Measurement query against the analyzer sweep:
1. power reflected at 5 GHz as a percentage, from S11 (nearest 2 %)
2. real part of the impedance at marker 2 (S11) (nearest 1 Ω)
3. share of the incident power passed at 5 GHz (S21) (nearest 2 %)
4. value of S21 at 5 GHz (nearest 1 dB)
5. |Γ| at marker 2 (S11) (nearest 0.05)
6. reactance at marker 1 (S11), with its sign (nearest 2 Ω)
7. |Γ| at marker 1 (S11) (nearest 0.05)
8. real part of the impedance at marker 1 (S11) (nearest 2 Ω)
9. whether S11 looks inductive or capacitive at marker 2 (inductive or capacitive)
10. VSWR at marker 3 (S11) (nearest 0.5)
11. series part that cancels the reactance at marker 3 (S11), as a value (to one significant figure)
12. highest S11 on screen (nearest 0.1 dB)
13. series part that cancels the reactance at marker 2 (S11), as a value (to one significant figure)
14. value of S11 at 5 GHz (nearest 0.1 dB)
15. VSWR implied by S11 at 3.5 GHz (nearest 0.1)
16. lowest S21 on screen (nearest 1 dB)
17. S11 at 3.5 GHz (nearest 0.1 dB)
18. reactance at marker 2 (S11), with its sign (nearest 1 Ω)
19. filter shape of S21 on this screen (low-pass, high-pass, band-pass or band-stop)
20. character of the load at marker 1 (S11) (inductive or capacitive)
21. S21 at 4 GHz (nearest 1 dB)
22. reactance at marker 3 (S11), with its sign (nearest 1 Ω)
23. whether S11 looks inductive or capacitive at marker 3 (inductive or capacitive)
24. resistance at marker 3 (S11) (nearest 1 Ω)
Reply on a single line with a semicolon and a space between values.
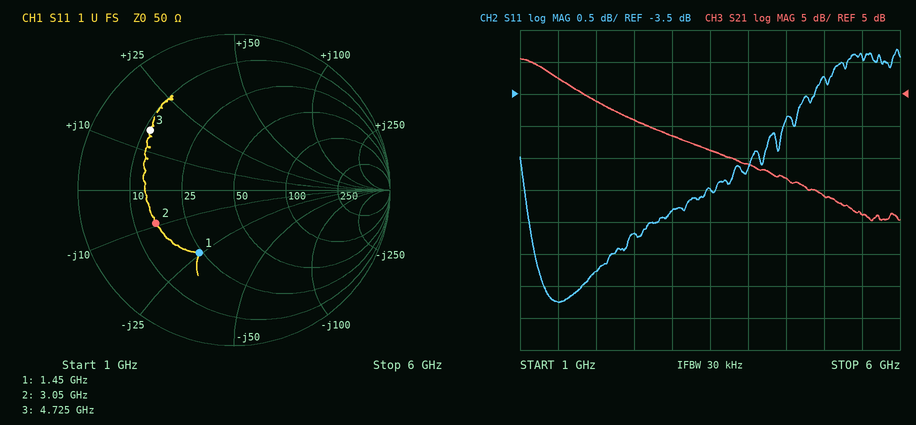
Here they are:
48 %; 15 Ω; 8 %; -11 dB; 0.55; -24 Ω; 0.45; 24 Ω; capacitive; 5.0; 2 pF; -2.8 dB; 500 pH; -3.2 dB; 3.6; -15 dB; -5.0 dB; -9 Ω; low-pass; capacitive; -6 dB; +15 Ω; inductive; 11 Ω
